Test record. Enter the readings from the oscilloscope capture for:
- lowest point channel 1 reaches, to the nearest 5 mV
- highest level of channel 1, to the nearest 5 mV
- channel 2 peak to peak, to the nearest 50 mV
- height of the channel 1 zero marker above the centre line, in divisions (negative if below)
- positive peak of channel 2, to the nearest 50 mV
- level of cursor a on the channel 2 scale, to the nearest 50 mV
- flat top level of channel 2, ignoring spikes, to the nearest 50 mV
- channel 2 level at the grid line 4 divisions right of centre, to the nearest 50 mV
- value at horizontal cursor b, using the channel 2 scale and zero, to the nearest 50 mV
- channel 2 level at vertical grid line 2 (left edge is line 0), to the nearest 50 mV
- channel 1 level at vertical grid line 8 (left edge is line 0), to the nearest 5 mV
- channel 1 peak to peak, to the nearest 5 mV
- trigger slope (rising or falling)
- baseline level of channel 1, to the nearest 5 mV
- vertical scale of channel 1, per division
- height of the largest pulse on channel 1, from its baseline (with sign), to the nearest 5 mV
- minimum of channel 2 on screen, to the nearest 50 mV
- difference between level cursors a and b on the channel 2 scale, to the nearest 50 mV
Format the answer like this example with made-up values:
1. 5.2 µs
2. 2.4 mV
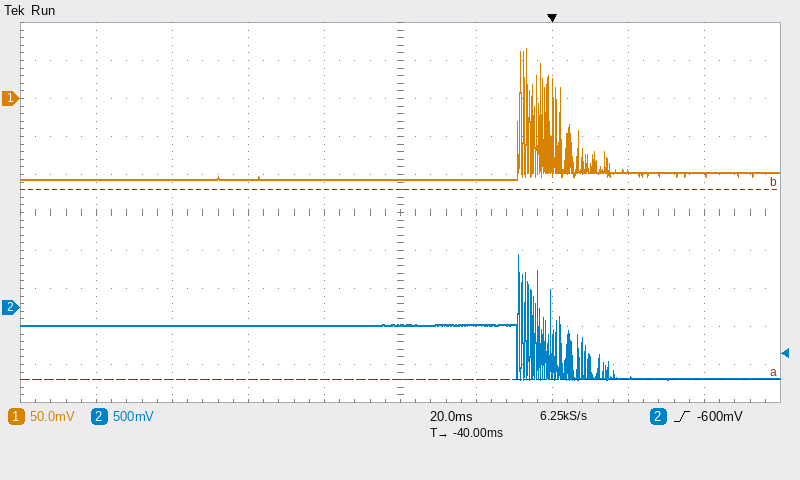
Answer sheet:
1. -105 mV
2. 65 mV
3. 1.65 V
4. +3.0 div
5. 700 mV
6. -950 mV
7. -250 mV
8. -950 mV
9. 1.55 V
10. -250 mV
11. -95 mV
12. 170 mV
13. rising
14. -105 mV
15. 50 mV
16. +170 mV
17. -950 mV
18. 2.50 V
